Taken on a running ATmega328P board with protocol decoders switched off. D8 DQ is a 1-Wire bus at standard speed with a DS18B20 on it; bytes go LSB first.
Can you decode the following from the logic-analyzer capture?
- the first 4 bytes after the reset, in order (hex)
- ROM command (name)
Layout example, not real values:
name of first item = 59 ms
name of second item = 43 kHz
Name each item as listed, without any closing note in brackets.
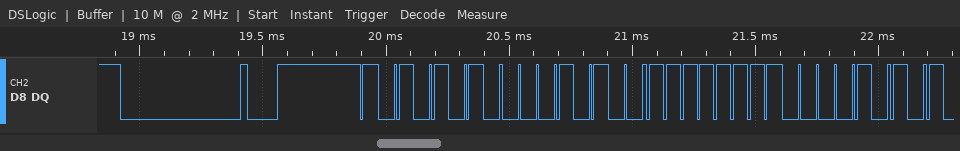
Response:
the first 4 bytes after the reset, in order = 55 28 FF 50
ROM command = Match ROM
